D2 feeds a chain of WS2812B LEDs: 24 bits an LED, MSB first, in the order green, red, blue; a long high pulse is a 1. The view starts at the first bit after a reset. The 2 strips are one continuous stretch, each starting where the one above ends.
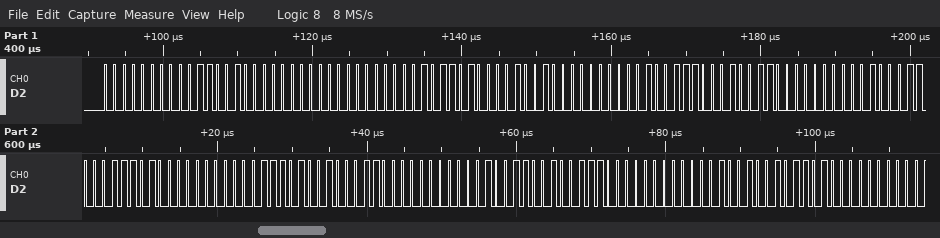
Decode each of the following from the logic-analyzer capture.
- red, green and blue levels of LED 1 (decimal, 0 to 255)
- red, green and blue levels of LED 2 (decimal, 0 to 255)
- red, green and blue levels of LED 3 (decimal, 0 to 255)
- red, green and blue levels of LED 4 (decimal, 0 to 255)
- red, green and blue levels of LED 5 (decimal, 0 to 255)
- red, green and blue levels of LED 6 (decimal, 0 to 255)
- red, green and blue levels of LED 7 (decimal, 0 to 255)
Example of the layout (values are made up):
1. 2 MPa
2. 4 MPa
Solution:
1. 50, 0, 0
2. 45, 0, 9
3. 39, 0, 19
4. 35, 0, 29
5. 29, 0, 35
6. 19, 0, 39
7. 9, 0, 45
